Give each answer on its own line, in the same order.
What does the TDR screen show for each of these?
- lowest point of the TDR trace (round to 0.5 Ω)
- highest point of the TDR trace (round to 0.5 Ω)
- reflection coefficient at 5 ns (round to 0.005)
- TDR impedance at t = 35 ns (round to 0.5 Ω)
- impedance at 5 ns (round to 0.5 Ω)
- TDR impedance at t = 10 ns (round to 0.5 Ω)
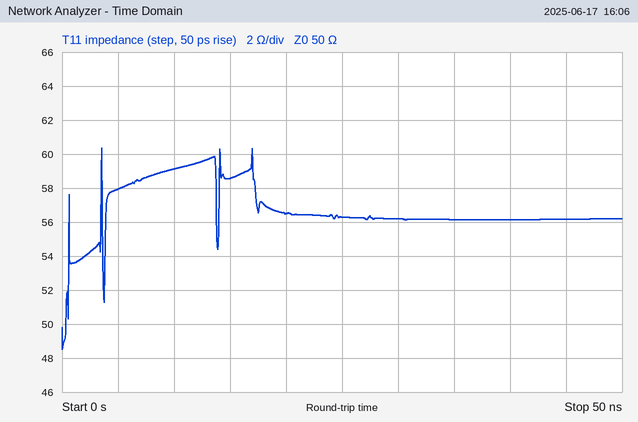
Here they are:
48.5 Ω
60.5 Ω
+0.075
56.0 Ω
58.0 Ω
59.0 Ω
